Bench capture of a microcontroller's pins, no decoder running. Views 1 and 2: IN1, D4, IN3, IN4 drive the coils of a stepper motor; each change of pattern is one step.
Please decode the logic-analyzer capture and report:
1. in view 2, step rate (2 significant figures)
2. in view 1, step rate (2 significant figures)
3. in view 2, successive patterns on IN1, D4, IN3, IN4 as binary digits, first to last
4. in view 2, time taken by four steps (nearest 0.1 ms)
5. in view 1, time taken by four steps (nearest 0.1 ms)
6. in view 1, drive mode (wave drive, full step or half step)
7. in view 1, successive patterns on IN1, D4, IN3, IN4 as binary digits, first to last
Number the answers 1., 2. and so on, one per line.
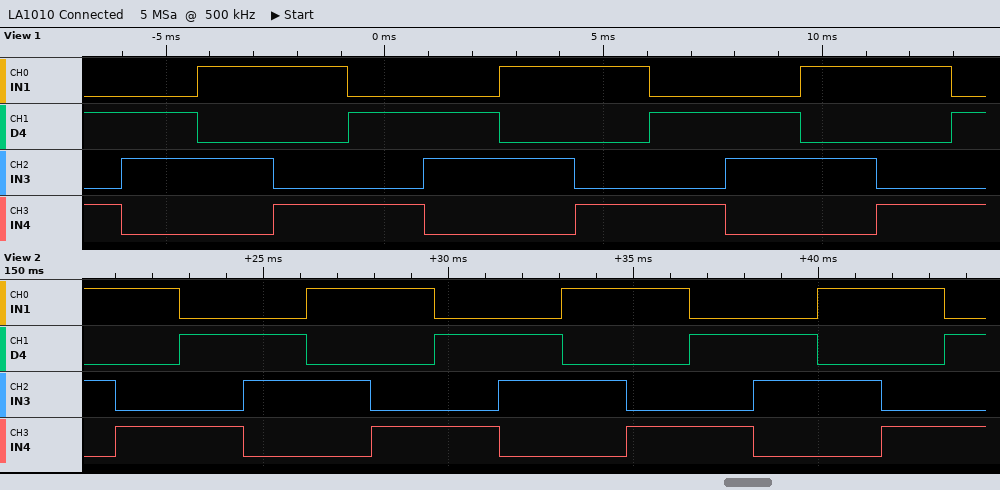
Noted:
1. 580 steps/s
2. 580 steps/s
3. 1010 1001 0101 0110 1010 1001 0101 0110 1010 1001 0101 0110 1010 1001 0101
4. 6.9 ms
5. 6.9 ms
6. full step
7. 0101 0110 1010 1001 0101 0110 1010 1001 0101 0110 1010 1001 0101
